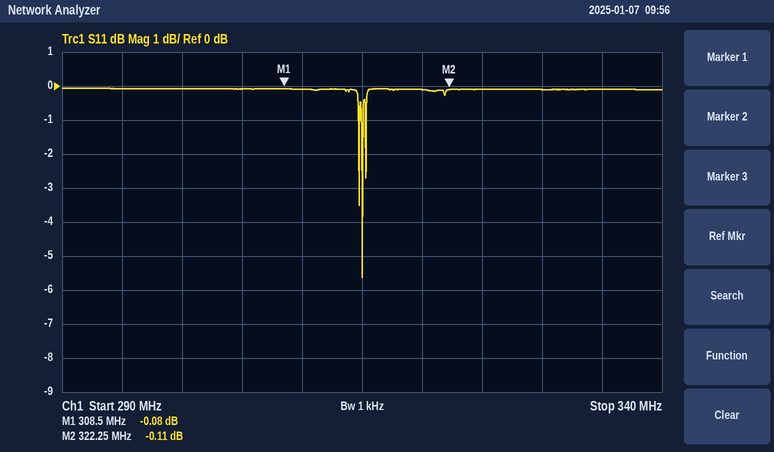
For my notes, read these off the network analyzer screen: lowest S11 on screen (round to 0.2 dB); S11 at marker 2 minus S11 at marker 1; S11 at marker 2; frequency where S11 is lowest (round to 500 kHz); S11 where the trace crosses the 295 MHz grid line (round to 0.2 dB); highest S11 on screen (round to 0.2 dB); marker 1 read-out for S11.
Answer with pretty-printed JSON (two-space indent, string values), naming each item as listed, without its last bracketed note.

{
  "lowest S11 on screen": "-5.6 dB",
  "S11 at marker 2 minus S11 at marker 1": "-0.03 dB",
  "S11 at marker 2": "-0.11 dB",
  "frequency where S11 is lowest": "315.0 MHz",
  "S11 where the trace crosses the 295 MHz grid line": "0.0 dB",
  "highest S11 on screen": "0.0 dB",
  "marker 1 read-out for S11": "-0.08 dB"
}
